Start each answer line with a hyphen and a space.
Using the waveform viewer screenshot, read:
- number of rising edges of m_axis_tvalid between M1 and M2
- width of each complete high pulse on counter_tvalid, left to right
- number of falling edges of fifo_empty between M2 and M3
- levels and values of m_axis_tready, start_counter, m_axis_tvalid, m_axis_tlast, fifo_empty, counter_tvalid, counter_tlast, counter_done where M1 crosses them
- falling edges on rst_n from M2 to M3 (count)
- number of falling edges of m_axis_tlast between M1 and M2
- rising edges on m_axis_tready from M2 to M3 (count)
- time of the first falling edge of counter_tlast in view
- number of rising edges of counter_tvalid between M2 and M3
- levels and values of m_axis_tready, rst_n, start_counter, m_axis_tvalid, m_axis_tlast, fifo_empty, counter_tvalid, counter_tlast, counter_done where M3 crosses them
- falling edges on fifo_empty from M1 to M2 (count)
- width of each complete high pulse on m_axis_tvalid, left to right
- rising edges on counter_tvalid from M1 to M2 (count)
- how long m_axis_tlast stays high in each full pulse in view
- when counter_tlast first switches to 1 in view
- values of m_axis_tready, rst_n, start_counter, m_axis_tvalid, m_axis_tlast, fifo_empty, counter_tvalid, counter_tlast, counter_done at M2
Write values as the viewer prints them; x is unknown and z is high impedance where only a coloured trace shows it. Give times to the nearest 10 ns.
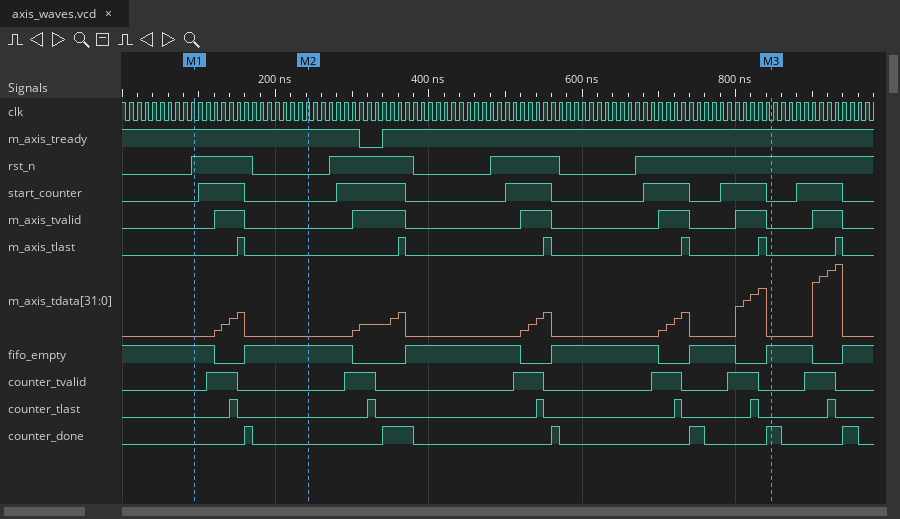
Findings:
- 1
- 40 ns, 40 ns, 40 ns, 40 ns, 40 ns, 40 ns
- 4
- m_axis_tready=1, start_counter=0, m_axis_tvalid=0, m_axis_tlast=0, fifo_empty=1, counter_tvalid=0, counter_tlast=0, counter_done=0
- 2
- 1
- 1
- 150 ns
- 4
- m_axis_tready=1, rst_n=1, start_counter=0, m_axis_tvalid=0, m_axis_tlast=0, fifo_empty=1, counter_tvalid=0, counter_tlast=0, counter_done=1
- 1
- 40 ns, 70 ns, 40 ns, 40 ns, 40 ns, 40 ns
- 1
- 10 ns, 10 ns, 10 ns, 10 ns, 10 ns, 10 ns
- 140 ns
- m_axis_tready=1, rst_n=0, start_counter=0, m_axis_tvalid=0, m_axis_tlast=0, fifo_empty=1, counter_tvalid=0, counter_tlast=0, counter_done=0
